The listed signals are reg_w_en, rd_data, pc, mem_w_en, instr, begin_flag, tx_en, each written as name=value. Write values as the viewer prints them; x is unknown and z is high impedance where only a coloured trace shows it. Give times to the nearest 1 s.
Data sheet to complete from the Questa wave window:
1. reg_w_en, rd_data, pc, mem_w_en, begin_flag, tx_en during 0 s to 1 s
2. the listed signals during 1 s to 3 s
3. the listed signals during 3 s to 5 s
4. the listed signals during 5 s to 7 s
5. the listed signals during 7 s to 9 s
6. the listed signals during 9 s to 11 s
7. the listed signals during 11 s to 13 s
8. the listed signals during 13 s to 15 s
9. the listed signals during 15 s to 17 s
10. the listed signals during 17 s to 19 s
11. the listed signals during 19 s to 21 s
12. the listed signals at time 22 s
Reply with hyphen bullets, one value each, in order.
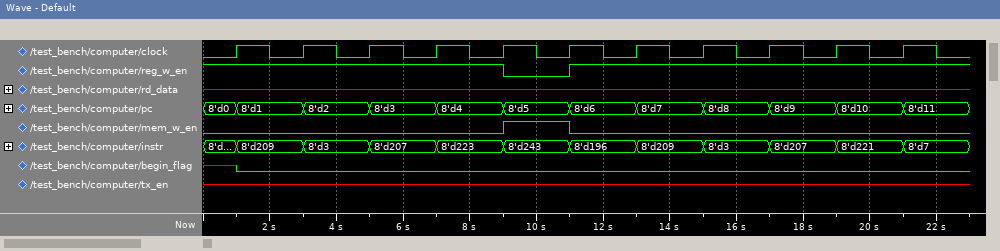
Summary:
- reg_w_en=1, rd_data=x, pc=8'd0, mem_w_en=0, begin_flag=x, tx_en=x
- reg_w_en=1, rd_data=x, pc=8'd1, mem_w_en=0, instr=8'd209, begin_flag=0, tx_en=x
- reg_w_en=1, rd_data=x, pc=8'd2, mem_w_en=0, instr=8'd3, begin_flag=0, tx_en=x
- reg_w_en=1, rd_data=x, pc=8'd3, mem_w_en=0, instr=8'd207, begin_flag=0, tx_en=x
- reg_w_en=1, rd_data=x, pc=8'd4, mem_w_en=0, instr=8'd223, begin_flag=0, tx_en=x
- reg_w_en=0, rd_data=x, pc=8'd5, mem_w_en=1, instr=8'd243, begin_flag=0, tx_en=x
- reg_w_en=1, rd_data=x, pc=8'd6, mem_w_en=0, instr=8'd196, begin_flag=0, tx_en=x
- reg_w_en=1, rd_data=x, pc=8'd7, mem_w_en=0, instr=8'd209, begin_flag=0, tx_en=x
- reg_w_en=1, rd_data=x, pc=8'd8, mem_w_en=0, instr=8'd3, begin_flag=0, tx_en=x
- reg_w_en=1, rd_data=x, pc=8'd9, mem_w_en=0, instr=8'd207, begin_flag=0, tx_en=x
- reg_w_en=1, rd_data=x, pc=8'd10, mem_w_en=0, instr=8'd221, begin_flag=0, tx_en=x
- reg_w_en=1, rd_data=x, pc=8'd11, mem_w_en=0, instr=8'd7, begin_flag=0, tx_en=x
